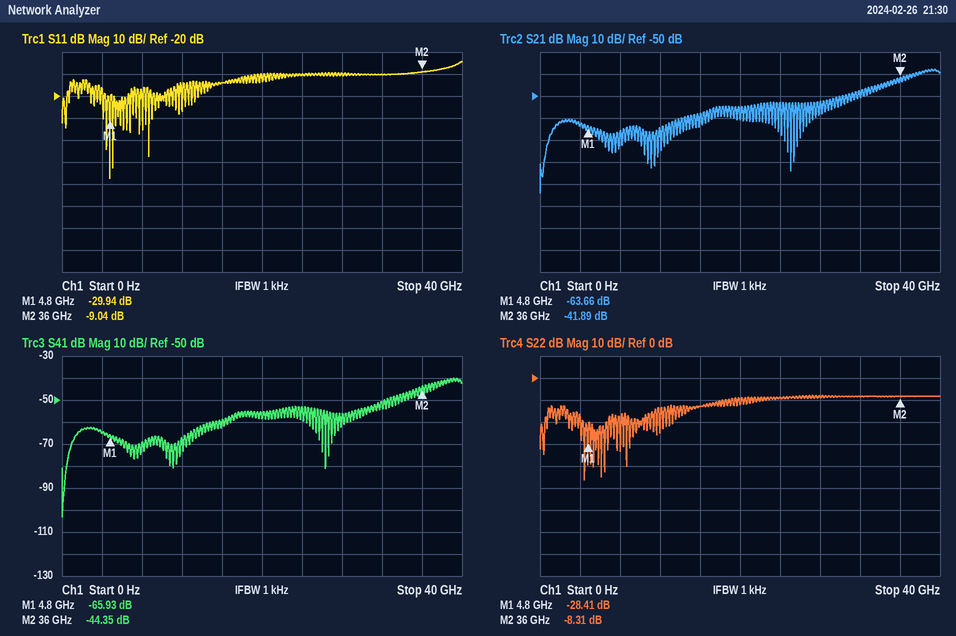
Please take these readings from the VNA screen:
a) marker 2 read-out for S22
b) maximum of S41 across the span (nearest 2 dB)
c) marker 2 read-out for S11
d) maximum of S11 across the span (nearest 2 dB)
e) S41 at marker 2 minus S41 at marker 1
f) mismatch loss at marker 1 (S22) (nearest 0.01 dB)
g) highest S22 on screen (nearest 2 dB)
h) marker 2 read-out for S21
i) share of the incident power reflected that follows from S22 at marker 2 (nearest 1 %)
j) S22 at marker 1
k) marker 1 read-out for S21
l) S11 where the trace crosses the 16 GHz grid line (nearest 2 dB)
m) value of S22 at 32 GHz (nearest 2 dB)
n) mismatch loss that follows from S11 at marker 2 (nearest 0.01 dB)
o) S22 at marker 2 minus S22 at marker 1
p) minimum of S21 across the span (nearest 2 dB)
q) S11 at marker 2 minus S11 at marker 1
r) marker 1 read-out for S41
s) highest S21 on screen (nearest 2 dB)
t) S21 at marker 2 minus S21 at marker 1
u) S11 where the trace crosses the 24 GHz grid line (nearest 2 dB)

-8.31 dB
-40 dB
-9.04 dB
-4 dB
21.58 dB
0.01 dB
-8 dB
-41.89 dB
15 %
-28.41 dB
-63.66 dB
-14 dB
-8 dB
0.58 dB
20.10 dB
-94 dB
20.90 dB
-65.93 dB
-38 dB
21.77 dB
-10 dB
